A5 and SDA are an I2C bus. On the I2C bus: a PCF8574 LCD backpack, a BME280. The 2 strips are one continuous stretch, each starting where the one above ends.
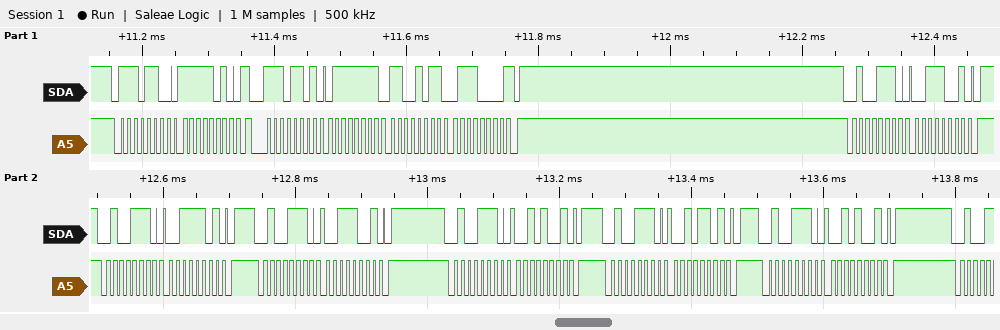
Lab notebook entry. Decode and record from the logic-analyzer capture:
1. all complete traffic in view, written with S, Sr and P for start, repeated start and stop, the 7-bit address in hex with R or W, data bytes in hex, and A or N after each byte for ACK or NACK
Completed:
S 76W A FA A Sr 76R A 7F A CB A 70 N P S 27W A 39 A P S 27W A 3D A P S 27W A 39 A P S 27W A 29 A P S 27W A 2D A P S 27W A 29 A P
